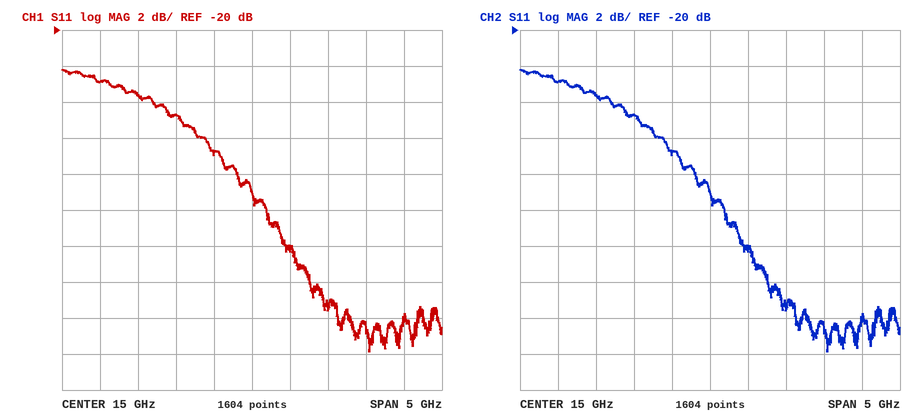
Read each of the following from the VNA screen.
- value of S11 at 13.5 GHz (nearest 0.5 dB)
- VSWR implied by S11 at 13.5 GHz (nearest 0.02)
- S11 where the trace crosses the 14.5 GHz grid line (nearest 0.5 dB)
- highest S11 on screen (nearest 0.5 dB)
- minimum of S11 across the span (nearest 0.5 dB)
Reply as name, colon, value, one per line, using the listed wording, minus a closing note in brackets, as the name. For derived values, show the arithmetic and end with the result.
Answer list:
value of S11 at 13.5 GHz: -23.5 dB
VSWR implied by S11 at 13.5 GHz: |Γ| = 10^(-23.5/20) = 0.0668; VSWR = (1 + 0.0668)/(1 − 0.0668) ≈ 1.14
S11 where the trace crosses the 14.5 GHz grid line: -27.0 dB
highest S11 on screen: -22.0 dB
minimum of S11 across the span: -38.0 dB
